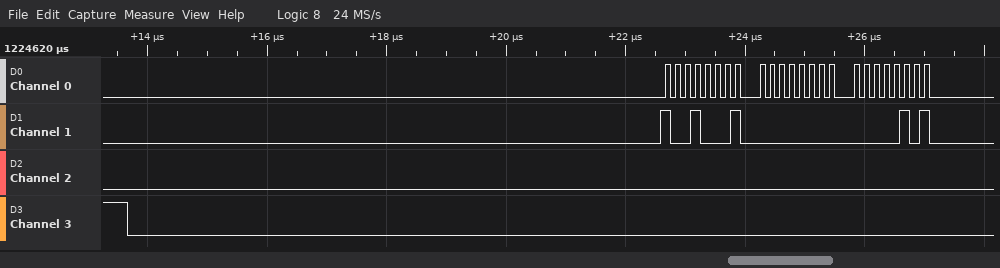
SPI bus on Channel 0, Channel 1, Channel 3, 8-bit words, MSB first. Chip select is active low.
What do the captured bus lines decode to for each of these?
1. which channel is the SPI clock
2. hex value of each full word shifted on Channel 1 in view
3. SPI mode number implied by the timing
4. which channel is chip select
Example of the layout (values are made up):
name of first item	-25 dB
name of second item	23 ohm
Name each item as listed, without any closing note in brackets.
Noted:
which channel is the SPI clock	Channel 0
hex value of each full word shifted on Channel 1 in view	91, 00, 05
SPI mode number implied by the timing	0
which channel is chip select	Channel 3
